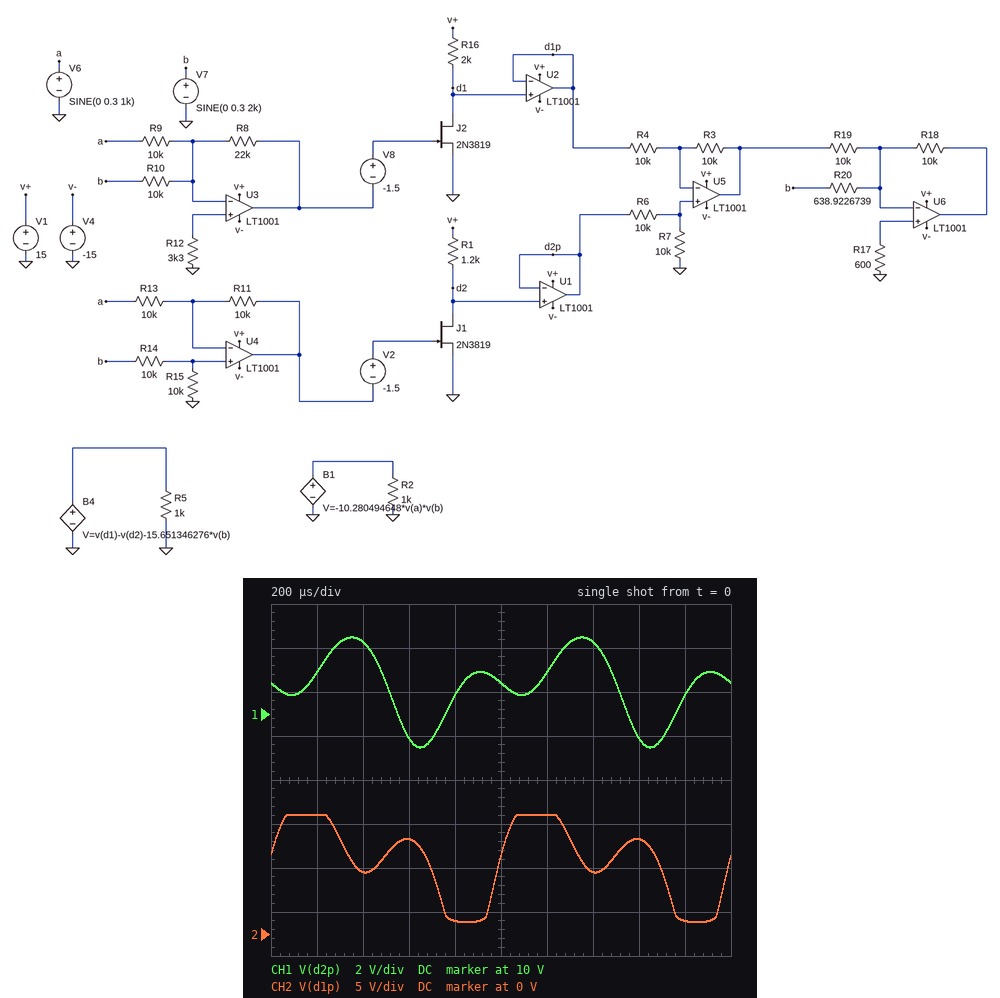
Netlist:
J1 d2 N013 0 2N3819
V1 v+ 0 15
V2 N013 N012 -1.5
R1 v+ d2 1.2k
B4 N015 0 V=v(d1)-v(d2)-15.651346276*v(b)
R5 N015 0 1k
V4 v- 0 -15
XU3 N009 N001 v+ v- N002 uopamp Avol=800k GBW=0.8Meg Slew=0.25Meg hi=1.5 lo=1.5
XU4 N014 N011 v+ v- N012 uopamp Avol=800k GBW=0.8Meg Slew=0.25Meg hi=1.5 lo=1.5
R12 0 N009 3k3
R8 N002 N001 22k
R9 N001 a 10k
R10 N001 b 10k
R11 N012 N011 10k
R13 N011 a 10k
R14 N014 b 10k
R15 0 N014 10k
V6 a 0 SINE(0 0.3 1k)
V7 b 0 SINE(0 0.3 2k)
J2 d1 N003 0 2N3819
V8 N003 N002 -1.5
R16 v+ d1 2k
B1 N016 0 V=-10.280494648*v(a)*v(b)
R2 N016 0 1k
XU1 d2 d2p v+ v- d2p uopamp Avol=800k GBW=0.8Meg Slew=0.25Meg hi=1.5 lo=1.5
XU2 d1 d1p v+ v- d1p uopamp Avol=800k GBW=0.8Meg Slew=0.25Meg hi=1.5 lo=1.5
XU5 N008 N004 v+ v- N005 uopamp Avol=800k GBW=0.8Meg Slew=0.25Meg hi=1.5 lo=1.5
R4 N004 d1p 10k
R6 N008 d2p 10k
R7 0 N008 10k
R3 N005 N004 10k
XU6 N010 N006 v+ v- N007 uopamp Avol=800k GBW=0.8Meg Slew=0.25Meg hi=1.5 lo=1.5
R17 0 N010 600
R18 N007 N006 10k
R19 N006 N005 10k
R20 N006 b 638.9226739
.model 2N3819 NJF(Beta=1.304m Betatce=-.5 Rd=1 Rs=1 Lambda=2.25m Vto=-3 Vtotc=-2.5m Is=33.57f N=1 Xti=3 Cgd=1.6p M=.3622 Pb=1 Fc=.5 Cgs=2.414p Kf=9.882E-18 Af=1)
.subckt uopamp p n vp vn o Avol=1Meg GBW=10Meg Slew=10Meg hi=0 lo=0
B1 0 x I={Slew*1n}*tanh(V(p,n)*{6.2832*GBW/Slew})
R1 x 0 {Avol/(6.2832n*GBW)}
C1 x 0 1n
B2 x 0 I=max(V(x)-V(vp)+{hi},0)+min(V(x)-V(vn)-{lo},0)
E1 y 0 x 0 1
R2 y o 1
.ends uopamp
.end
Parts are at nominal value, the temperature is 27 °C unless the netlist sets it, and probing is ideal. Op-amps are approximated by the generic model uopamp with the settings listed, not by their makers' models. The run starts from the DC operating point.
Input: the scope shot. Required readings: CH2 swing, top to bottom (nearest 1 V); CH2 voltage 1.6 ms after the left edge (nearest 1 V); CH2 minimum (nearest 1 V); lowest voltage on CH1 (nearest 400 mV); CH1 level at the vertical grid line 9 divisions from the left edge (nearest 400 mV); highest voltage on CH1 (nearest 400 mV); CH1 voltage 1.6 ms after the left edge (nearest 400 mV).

12 V
11 V
1 V
8.4 V
10.8 V
13.6 V
8.8 V
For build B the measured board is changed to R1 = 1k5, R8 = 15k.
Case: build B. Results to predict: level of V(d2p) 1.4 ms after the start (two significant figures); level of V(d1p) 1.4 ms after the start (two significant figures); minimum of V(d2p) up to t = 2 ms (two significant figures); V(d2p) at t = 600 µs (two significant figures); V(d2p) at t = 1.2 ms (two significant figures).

13 V
7.7 V
6.9 V
7.4 V
11 V
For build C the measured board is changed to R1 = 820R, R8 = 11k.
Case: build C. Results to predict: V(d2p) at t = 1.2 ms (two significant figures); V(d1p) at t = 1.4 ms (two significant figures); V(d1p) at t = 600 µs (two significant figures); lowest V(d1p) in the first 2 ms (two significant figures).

13 V
8.1 V
9.9 V
3.7 V
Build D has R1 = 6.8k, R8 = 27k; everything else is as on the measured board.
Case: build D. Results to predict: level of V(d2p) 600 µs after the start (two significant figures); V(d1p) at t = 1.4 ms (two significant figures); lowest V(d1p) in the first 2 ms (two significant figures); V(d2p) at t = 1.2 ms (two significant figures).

480 mV
6.5 V
1.1 V
810 mV
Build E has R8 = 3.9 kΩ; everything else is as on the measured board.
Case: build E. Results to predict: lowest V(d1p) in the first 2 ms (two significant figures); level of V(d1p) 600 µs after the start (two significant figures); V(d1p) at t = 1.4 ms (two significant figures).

7.3 V
9.4 V
8.7 V
